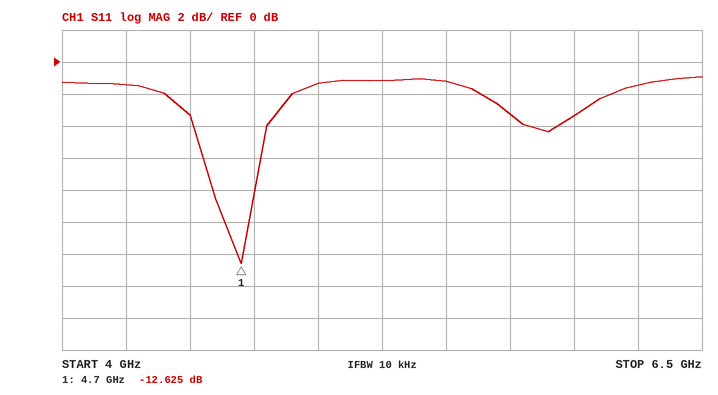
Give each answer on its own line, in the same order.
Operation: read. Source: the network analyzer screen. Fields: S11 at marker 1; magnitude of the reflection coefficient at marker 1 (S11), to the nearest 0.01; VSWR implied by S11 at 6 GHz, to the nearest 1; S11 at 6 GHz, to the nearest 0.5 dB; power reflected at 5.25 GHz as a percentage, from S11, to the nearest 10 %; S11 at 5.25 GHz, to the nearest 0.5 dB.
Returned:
-12.625 dB
0.23
5
-3.5 dB
80 %
-1.0 dB
